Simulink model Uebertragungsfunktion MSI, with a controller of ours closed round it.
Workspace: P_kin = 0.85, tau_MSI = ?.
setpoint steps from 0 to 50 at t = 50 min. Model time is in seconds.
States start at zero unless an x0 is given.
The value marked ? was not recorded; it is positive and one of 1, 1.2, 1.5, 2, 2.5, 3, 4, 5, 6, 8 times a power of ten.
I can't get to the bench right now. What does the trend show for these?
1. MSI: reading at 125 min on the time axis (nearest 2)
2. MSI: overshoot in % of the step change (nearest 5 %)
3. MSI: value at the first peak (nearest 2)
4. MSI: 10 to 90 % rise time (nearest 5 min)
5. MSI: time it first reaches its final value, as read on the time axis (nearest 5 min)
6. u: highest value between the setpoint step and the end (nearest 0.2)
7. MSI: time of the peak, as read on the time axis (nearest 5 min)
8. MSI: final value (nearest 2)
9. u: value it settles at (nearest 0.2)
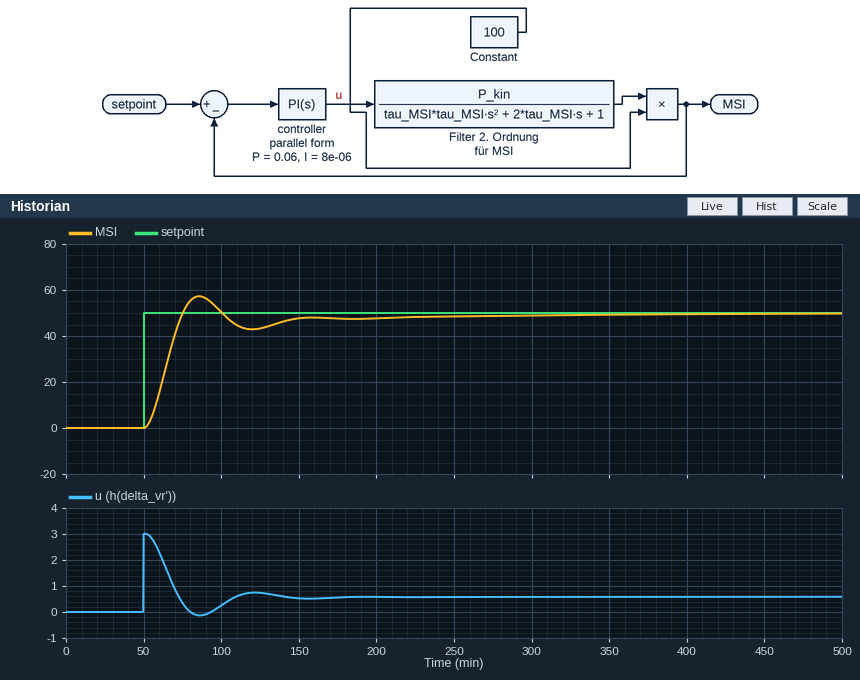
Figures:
44
15 %
58
15 min
75 min
3.0
85 min
50
0.6
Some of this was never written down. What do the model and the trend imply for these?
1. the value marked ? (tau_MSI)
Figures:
1500
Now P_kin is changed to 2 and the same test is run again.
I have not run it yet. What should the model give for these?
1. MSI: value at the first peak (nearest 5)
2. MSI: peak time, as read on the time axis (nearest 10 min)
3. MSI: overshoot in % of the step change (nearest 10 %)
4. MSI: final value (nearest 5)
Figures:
70
70 min
40 %
50
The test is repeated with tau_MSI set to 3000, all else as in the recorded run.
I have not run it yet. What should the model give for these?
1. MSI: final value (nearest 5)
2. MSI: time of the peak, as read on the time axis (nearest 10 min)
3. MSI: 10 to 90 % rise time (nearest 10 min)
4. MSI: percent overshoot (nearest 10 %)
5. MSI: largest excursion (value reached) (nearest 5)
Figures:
50
120 min
30 min
20 %
60
